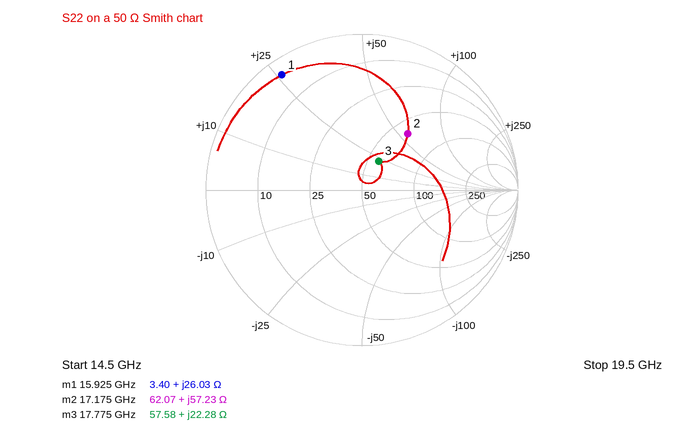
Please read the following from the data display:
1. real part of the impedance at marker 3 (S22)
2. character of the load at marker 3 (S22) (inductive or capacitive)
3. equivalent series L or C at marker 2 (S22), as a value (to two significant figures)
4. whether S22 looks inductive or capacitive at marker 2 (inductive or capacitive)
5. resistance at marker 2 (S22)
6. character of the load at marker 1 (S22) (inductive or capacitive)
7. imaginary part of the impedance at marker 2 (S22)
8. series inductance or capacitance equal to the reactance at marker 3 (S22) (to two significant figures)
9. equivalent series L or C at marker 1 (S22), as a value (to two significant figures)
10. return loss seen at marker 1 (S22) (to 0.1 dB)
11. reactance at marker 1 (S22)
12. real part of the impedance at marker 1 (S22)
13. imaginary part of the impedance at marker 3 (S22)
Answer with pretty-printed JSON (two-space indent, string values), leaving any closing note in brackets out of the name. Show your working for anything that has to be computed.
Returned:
{
  "real part of the impedance at marker 3": "57.58 Ω",
  "character of the load at marker 3 (S22)": "inductive",
  "equivalent series L or C at marker 2 (S22), as a value": "L = 57.23 Ω/(2π × 17.175 GHz) ≈ 530 pH",
  "whether S22 looks inductive or capacitive at marker 2": "inductive",
  "resistance at marker 2": "62.07 Ω",
  "character of the load at marker 1 (S22)": "inductive",
  "imaginary part of the impedance at marker 2": "+57.23 Ω",
  "series inductance or capacitance equal to the reactance at marker 3 (S22)": "L = 22.28 Ω/(2π × 17.775 GHz) ≈ 199 pH, so 200 pH to two significant figures",
  "equivalent series L or C at marker 1 (S22), as a value": "L = 26.03 Ω/(2π × 15.925 GHz) ≈ 260 pH",
  "return loss seen at marker 1 (S22)": "0.9 dB",
  "reactance at marker 1": "+26.03 Ω",
  "real part of the impedance at marker 1": "3.40 Ω",
  "imaginary part of the impedance at marker 3": "+22.28 Ω"
}
